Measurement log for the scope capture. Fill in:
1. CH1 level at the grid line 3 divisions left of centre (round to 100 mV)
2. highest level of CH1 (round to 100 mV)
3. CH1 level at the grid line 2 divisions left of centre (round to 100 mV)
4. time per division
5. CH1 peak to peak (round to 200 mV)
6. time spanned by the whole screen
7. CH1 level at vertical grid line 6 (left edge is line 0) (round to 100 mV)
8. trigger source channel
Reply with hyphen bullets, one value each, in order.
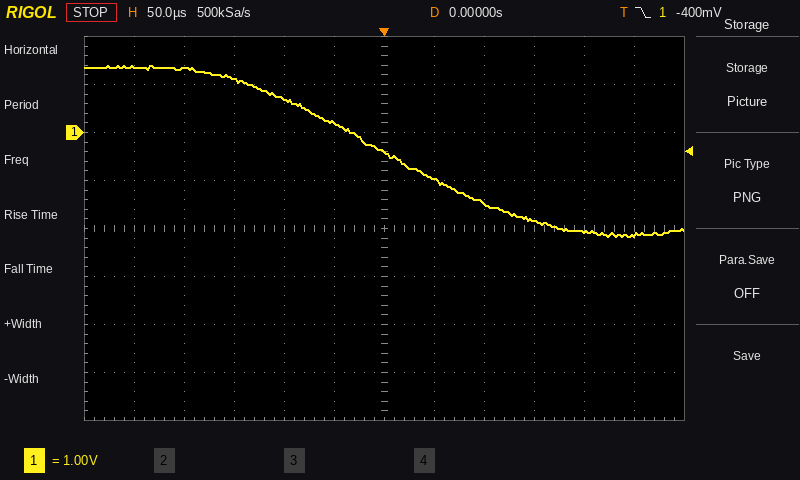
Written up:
- 1.1 V
- 1.4 V
- 700 mV
- 50 µs
- 3.6 V
- 600 µs
- -400 mV
- CH1
